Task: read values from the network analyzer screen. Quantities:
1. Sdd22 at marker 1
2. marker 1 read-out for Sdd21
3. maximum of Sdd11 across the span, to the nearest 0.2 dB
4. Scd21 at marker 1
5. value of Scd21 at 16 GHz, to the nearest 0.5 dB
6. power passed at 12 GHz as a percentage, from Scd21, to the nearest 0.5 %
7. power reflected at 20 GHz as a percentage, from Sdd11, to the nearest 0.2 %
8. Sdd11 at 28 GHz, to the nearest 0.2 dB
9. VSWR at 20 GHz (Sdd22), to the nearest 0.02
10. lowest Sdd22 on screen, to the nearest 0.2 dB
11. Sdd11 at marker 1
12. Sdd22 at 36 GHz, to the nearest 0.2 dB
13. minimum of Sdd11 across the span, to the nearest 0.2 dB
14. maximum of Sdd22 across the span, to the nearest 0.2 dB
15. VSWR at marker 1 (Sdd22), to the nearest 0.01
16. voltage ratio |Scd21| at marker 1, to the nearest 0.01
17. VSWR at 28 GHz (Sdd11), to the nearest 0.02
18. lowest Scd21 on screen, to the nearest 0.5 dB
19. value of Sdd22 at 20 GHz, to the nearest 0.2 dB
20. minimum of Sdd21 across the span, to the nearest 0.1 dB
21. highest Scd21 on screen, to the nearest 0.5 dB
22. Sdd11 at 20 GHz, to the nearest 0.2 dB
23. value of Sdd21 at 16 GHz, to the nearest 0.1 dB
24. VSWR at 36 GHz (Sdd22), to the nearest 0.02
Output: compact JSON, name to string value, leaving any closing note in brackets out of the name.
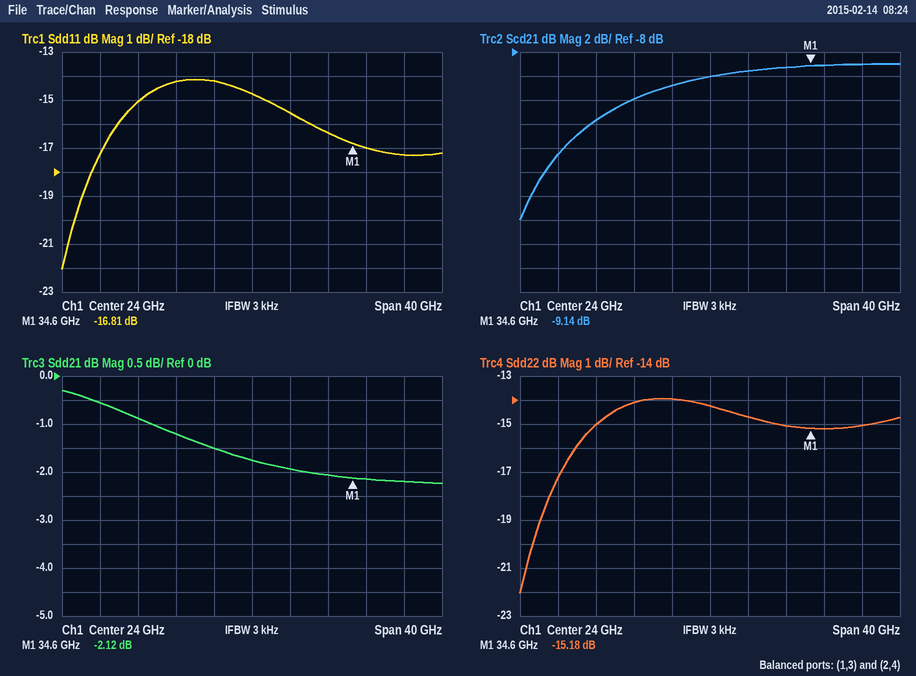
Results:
{"Sdd22 at marker 1": "-15.18 dB", "marker 1 read-out for Sdd21": "-2.12 dB", "maximum of Sdd11 across the span, to the nearest 0.2 dB": "-14.2 dB", "Scd21 at marker 1": "-9.14 dB", "value of Scd21 at 16 GHz, to the nearest 0.5 dB": "-12.0 dB", "power passed at 12 GHz as a percentage, from Scd21, to the nearest 0.5 %": "4.5 %", "power reflected at 20 GHz as a percentage, from Sdd11, to the nearest 0.2 %": "3.8 %", "Sdd11 at 28 GHz, to the nearest 0.2 dB": "-15.6 dB", "VSWR at 20 GHz (Sdd22), to the nearest 0.02": "1.50", "lowest Sdd22 on screen, to the nearest 0.2 dB": "-22.0 dB", "Sdd11 at marker 1": "-16.81 dB", "Sdd22 at 36 GHz, to the nearest 0.2 dB": "-15.2 dB", "minimum of Sdd11 across the span, to the nearest 0.2 dB": "-22.0 dB", "maximum of Sdd22 across the span, to the nearest 0.2 dB": "-14.0 dB", "VSWR at marker 1 (Sdd22), to the nearest 0.01": "1.42", "voltage ratio |Scd21| at marker 1, to the nearest 0.01": "0.35", "VSWR at 28 GHz (Sdd11), to the nearest 0.02": "1.40", "lowest Scd21 on screen, to the nearest 0.5 dB": "-22.0 dB", "value of Sdd22 at 20 GHz, to the nearest 0.2 dB": "-14.0 dB", "minimum of Sdd21 across the span, to the nearest 0.1 dB": "-2.2 dB", "highest Scd21 on screen, to the nearest 0.5 dB": "-9.0 dB", "Sdd11 at 20 GHz, to the nearest 0.2 dB": "-14.2 dB", "value of Sdd21 at 16 GHz, to the nearest 0.1 dB": "-1.2 dB", "VSWR at 36 GHz (Sdd22), to the nearest 0.02": "1.42"}
